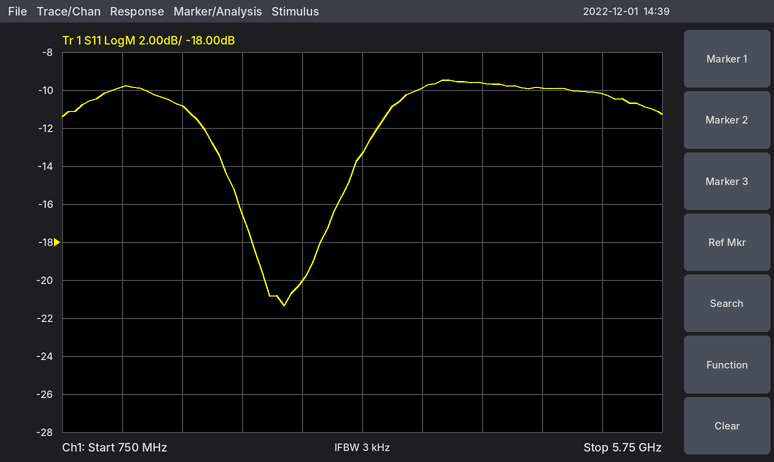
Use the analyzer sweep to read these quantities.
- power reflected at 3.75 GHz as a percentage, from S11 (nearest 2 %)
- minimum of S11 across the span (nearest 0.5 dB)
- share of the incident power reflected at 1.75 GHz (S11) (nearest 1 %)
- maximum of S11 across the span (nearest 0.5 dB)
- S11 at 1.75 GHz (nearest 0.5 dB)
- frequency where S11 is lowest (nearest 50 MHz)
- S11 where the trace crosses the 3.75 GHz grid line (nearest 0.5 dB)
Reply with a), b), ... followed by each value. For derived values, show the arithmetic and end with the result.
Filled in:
a) 10^(-10/10) ≈ 10 %
b) -21.5 dB
c) 10^(-11/10) ≈ 8 %
d) -9.5 dB
e) -11.0 dB
f) 2.60 GHz
g) -10.0 dB
